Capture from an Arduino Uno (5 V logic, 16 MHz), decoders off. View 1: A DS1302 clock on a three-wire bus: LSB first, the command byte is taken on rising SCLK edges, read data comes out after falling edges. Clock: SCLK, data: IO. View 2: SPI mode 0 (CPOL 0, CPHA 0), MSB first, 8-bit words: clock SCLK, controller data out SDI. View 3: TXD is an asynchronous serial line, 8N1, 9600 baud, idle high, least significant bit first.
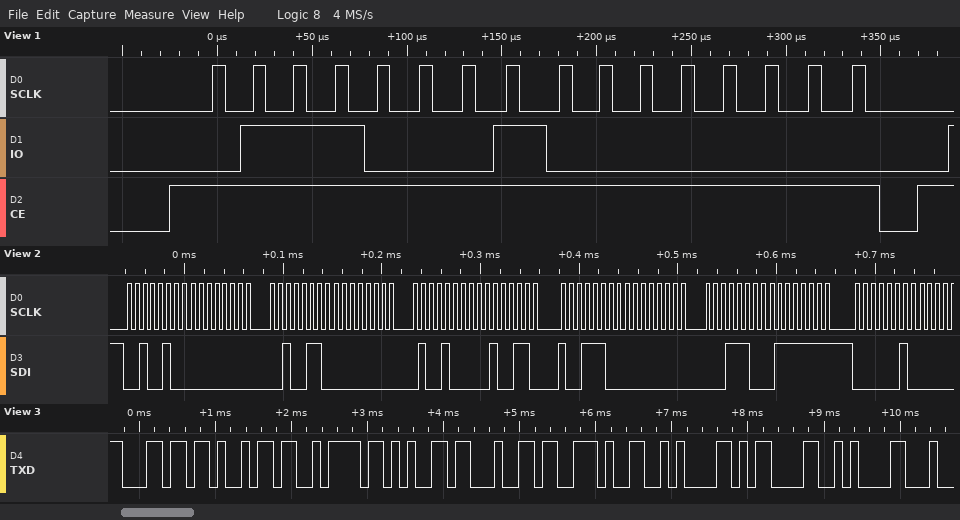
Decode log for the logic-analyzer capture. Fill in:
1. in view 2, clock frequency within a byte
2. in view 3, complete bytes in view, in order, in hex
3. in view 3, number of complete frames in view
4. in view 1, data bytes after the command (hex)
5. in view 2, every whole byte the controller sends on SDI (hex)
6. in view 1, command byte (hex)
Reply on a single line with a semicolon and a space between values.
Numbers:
125 kHz; 6C 69 7A 65 64 2E 0A 0D 0A; 9; 00; 24 00 26 00 48 26 9C 00 1C 7F 02; 0x8E
